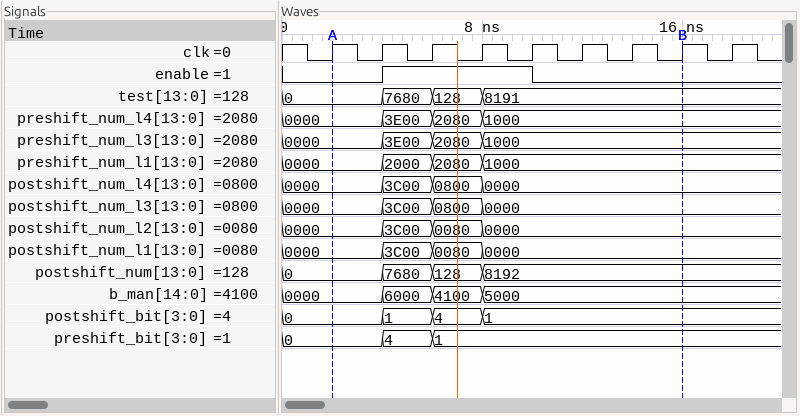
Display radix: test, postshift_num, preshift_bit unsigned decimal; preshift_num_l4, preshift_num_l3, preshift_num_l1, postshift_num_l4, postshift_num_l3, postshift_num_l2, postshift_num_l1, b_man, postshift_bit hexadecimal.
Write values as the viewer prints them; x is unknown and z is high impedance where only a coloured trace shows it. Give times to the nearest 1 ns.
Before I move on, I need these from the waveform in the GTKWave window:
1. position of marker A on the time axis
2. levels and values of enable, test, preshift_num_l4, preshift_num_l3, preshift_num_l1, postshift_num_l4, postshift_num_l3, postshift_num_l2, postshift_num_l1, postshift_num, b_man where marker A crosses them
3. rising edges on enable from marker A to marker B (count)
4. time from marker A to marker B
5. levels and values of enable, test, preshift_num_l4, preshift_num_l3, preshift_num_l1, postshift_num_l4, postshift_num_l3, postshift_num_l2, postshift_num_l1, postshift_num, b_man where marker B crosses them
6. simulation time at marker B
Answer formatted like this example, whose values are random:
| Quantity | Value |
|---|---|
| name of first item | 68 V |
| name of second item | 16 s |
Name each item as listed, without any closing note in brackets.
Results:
| Quantity | Value |
|---|---|
| position of marker A on the time axis | 2 ns |
| levels and values of enable, test, preshift_num_l4, preshift_num_l3, preshift_num_l1, postshift_num_l4, postshift_num_l3, postshift_num_l2, postshift_num_l1, postshift_num, b_man where marker A crosses them | enable=0, test=0, preshift_num_l4=0000, preshift_num_l3=0000, preshift_num_l1=0000, postshift_num_l4=0000, postshift_num_l3=0000, postshift_num_l2=0000, postshift_num_l1=0000, postshift_num=0, b_man=0000 |
| rising edges on enable from marker A to marker B | 1 |
| time from marker A to marker B | 14 ns |
| levels and values of enable, test, preshift_num_l4, preshift_num_l3, preshift_num_l1, postshift_num_l4, postshift_num_l3, postshift_num_l2, postshift_num_l1, postshift_num, b_man where marker B crosses them | enable=0, test=8191, preshift_num_l4=1000, preshift_num_l3=1000, preshift_num_l1=1000, postshift_num_l4=0000, postshift_num_l3=0000, postshift_num_l2=0000, postshift_num_l1=0000, postshift_num=8192, b_man=5000 |
| simulation time at marker B | 16 ns |
